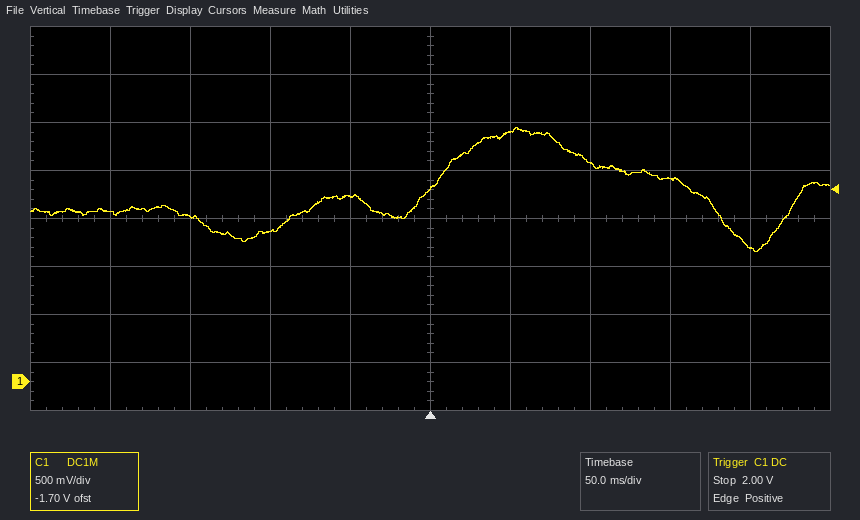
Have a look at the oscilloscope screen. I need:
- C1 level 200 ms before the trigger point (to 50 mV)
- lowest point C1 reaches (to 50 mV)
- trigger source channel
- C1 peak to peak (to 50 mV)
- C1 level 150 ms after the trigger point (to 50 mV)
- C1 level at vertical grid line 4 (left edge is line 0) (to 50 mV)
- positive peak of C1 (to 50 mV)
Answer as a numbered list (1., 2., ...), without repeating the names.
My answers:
1. 1.75 V
2. 1.35 V
3. C1
4. 1.30 V
5. 2.10 V
6. 1.95 V
7. 2.65 V
